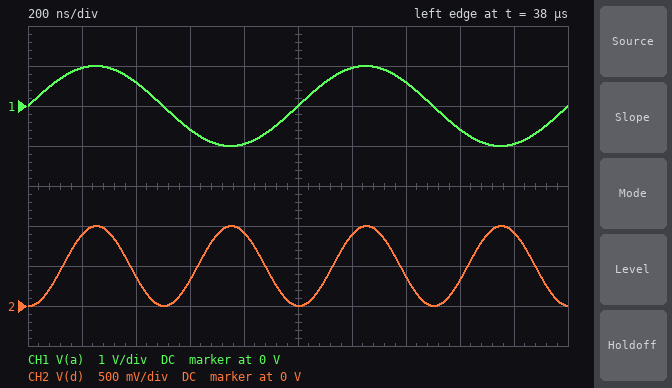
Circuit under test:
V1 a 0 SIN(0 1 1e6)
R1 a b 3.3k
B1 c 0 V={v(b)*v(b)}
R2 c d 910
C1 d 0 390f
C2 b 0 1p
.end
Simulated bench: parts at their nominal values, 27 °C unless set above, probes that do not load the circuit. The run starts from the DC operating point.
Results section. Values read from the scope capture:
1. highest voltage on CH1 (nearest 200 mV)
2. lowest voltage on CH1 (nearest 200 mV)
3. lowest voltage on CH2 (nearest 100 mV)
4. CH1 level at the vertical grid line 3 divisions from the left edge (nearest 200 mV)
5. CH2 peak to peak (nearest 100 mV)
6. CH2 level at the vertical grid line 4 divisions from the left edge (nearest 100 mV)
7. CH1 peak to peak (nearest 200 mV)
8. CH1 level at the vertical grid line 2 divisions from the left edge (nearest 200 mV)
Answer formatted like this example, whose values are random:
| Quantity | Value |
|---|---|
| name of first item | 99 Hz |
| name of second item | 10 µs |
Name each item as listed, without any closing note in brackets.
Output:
| Quantity | Value |
|---|---|
| highest voltage on CH1 | 1.0 V |
| lowest voltage on CH1 | -1.0 V |
| lowest voltage on CH2 | 0 V |
| CH1 level at the vertical grid line 3 divisions from the left edge | -600 mV |
| CH2 peak to peak | 1.0 V |
| CH2 level at the vertical grid line 4 divisions from the left edge | 900 mV |
| CH1 peak to peak | 2.0 V |
| CH1 level at the vertical grid line 2 divisions from the left edge | 600 mV |
